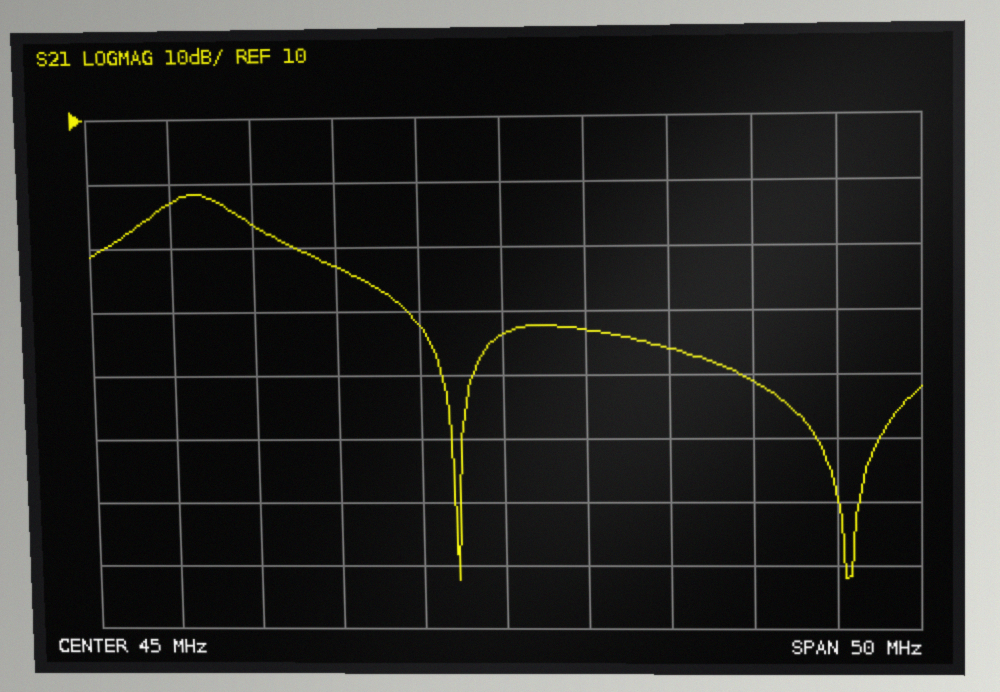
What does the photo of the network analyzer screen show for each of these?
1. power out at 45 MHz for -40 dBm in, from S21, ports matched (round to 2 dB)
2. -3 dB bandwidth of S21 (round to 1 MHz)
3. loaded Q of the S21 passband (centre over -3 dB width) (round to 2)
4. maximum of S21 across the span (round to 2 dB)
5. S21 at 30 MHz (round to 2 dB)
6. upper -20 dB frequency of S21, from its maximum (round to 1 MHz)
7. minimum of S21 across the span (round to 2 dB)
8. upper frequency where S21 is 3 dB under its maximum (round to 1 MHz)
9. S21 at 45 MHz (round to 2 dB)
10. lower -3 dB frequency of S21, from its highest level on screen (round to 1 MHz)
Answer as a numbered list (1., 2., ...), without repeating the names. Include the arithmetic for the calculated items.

1. -40 dBm + (-24 dB) = -64 dBm
2. 29 MHz − 24 MHz = 5 MHz
3. 26.5 MHz / 5 MHz ≈ 5.30, so 6 to the nearest 2
4. -2 dB
5. -6 dB
6. 40 MHz
7. -62 dB
8. 29 MHz
9. -24 dB
10. 24 MHz
